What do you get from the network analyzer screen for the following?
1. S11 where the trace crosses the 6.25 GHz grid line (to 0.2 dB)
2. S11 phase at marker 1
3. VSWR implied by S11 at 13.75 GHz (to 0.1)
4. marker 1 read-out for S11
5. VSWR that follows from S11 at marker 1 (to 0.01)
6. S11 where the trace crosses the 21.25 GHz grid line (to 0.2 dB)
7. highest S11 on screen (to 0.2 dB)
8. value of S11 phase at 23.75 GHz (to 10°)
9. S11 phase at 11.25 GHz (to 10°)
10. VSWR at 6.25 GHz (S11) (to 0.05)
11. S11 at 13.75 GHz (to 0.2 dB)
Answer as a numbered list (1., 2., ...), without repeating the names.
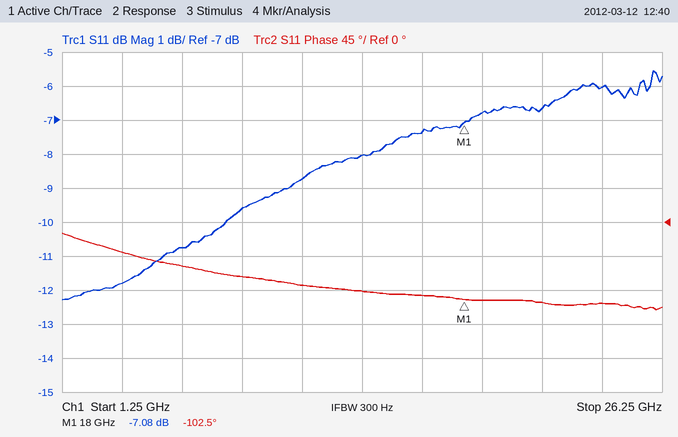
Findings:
1. -10.8 dB
2. -102.5°
3. 2.3
4. -7.08 dB
5. 2.59
6. -6.6 dB
7. -5.6 dB
8. -110°
9. -80°
10. 1.80
11. -8.0 dB
